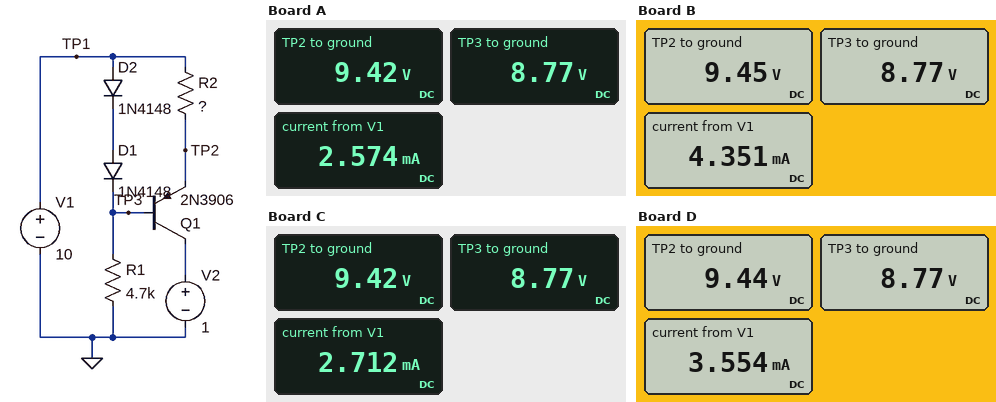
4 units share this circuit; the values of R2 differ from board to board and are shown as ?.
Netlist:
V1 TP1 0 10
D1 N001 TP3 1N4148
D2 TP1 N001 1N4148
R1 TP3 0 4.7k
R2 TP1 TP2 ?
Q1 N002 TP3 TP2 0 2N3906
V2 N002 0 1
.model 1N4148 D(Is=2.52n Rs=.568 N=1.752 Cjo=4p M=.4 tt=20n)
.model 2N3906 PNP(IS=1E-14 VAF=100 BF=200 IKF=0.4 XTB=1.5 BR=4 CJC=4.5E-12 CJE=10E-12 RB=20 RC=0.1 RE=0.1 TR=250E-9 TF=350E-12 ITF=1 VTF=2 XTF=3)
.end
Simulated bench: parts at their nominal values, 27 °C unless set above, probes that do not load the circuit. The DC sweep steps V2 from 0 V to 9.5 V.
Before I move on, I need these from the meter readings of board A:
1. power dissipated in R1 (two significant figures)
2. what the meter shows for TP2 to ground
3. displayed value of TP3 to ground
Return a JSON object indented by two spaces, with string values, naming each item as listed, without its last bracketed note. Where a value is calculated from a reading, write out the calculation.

{
  "power dissipated in R1": "(8.77 V)^2 / 4.7 kΩ = 16 mW",
  "what the meter shows for TP2 to ground": "9.42 V",
  "displayed value of TP3 to ground": "8.77 V"
}
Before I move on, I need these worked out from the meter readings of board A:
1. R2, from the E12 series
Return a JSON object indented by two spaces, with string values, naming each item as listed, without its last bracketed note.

{
  "R2, from the E12 series": "820 Ω"
}
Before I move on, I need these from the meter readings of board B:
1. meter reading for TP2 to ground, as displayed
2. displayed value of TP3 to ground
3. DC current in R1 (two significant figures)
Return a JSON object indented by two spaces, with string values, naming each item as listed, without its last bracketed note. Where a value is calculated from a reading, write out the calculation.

{
  "meter reading for TP2 to ground, as displayed": "9.45 V",
  "displayed value of TP3 to ground": "8.77 V",
  "DC current in R1": "(8.77 V) / 4.7 kΩ = 1.9 mA"
}
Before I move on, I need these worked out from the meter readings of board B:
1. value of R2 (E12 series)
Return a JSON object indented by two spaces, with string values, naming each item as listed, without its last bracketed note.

{
  "value of R2": "220 Ω"
}
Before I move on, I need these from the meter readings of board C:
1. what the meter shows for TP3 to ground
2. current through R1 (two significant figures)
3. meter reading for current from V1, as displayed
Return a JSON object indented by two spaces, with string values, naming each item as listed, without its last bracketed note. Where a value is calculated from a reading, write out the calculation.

{
  "what the meter shows for TP3 to ground": "8.77 V",
  "current through R1": "(8.77 V) / 4.7 kΩ = 1.9 mA",
  "meter reading for current from V1, as displayed": "2.712 mA"
}
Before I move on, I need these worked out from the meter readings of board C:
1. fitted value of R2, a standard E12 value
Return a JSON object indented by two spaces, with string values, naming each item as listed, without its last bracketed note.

{
  "fitted value of R2, a standard E12 value": "680 Ω"
}
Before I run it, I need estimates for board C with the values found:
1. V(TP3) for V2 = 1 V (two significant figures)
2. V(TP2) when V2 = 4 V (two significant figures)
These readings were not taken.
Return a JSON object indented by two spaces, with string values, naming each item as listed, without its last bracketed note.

{
  "V(TP3) for V2 = 1 V": "8.8 V",
  "V(TP2) when V2 = 4 V": "9.4 V"
}
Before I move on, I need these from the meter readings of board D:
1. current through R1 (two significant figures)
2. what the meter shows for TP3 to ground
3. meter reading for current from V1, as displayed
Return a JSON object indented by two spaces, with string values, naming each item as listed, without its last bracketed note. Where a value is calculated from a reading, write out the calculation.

{
  "current through R1": "(8.77 V) / 4.7 kΩ = 1.9 mA",
  "what the meter shows for TP3 to ground": "8.77 V",
  "meter reading for current from V1, as displayed": "3.554 mA"
}
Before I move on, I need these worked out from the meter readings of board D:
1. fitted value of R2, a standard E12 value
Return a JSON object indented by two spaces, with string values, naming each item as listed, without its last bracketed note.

{
  "fitted value of R2, a standard E12 value": "330 Ω"
}
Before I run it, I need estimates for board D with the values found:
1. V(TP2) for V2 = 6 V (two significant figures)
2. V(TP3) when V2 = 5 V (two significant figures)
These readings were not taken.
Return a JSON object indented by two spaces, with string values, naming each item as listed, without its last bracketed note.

{
  "V(TP2) for V2 = 6 V": "9.4 V",
  "V(TP3) when V2 = 5 V": "8.8 V"
}
